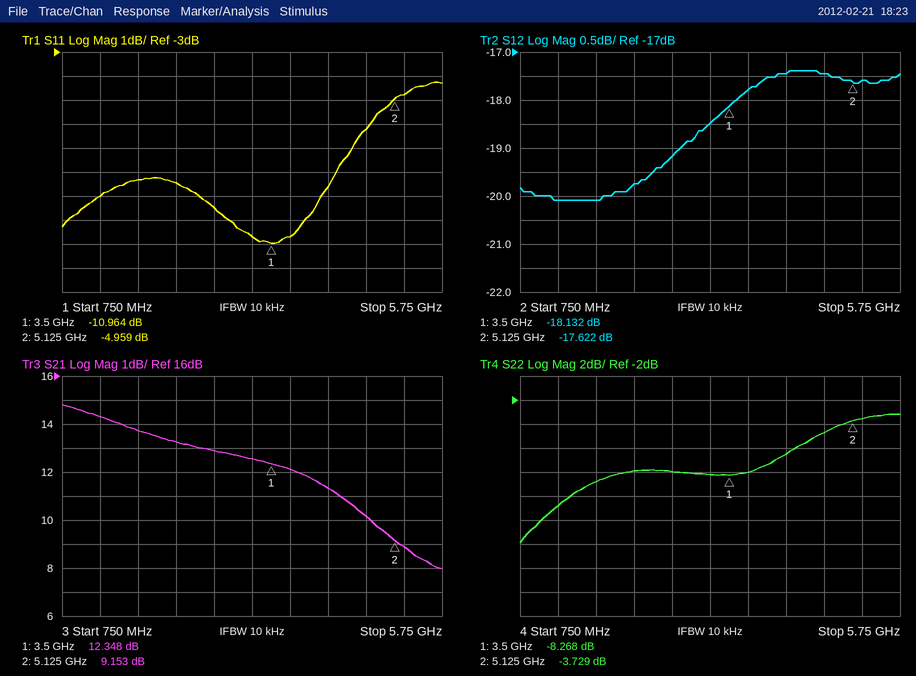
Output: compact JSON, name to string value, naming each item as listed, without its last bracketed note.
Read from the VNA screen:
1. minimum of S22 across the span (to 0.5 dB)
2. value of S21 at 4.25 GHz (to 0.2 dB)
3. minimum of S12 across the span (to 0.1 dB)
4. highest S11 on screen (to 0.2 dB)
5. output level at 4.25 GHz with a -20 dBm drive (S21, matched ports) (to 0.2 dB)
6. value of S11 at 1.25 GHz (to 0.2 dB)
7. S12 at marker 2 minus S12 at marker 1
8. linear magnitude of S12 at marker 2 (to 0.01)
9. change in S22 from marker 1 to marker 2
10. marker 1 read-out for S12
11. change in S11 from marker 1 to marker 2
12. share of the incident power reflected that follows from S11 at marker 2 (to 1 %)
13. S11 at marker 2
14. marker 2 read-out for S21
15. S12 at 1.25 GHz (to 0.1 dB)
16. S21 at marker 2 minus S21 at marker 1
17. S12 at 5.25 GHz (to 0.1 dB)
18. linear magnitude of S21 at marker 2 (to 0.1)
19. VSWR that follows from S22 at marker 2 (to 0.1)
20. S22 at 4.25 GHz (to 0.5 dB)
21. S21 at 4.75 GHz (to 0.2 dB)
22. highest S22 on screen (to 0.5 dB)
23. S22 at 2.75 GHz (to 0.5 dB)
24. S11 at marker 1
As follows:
{"minimum of S22 across the span": "-14.0 dB", "value of S21 at 4.25 GHz": "11.4 dB", "minimum of S12 across the span": "-20.1 dB", "highest S11 on screen": "-4.2 dB", "output level at 4.25 GHz with a -20 dBm drive (S21, matched ports)": "-8.6 dBm", "value of S11 at 1.25 GHz": "-9.0 dB", "S12 at marker 2 minus S12 at marker 1": "0.510 dB", "linear magnitude of S12 at marker 2": "0.13", "change in S22 from marker 1 to marker 2": "4.539 dB", "marker 1 read-out for S12": "-18.132 dB", "change in S11 from marker 1 to marker 2": "6.005 dB", "share of the incident power reflected that follows from S11 at marker 2": "32 %", "S11 at marker 2": "-4.959 dB", "marker 2 read-out for S21": "9.153 dB", "S12 at 1.25 GHz": "-20.1 dB", "S21 at marker 2 minus S21 at marker 1": "-3.195 dB", "S12 at 5.25 GHz": "-17.6 dB", "linear magnitude of S21 at marker 2": "2.9", "VSWR that follows from S22 at marker 2": "4.7", "S22 at 4.25 GHz": "-6.5 dB", "S21 at 4.75 GHz": "10.2 dB", "highest S22 on screen": "-3.0 dB", "S22 at 2.75 GHz": "-8.0 dB", "S11 at marker 1": "-10.964 dB"}
